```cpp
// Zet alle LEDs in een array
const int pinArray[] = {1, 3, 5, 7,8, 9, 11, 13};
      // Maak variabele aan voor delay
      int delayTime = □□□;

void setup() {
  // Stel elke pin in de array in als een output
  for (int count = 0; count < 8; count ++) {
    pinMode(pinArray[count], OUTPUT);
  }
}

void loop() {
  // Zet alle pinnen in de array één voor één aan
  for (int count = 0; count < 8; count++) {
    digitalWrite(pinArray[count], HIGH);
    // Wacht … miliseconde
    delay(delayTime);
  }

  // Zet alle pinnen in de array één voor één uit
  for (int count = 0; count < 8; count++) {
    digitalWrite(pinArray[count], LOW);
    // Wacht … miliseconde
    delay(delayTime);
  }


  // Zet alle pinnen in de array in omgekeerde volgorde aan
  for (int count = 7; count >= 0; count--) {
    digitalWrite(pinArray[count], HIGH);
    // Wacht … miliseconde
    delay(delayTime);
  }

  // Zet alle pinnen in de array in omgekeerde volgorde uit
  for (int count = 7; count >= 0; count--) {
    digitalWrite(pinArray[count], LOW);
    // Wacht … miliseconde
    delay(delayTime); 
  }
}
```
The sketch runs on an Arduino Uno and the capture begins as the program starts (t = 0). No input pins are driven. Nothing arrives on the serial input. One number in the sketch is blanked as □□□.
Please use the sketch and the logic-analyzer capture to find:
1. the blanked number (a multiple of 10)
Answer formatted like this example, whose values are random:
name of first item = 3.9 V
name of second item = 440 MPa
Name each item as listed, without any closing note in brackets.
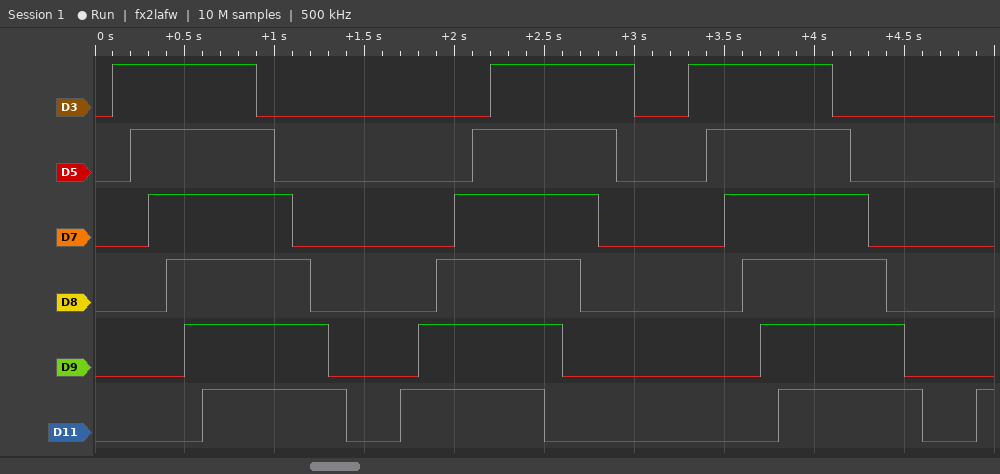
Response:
the blanked number = 100
